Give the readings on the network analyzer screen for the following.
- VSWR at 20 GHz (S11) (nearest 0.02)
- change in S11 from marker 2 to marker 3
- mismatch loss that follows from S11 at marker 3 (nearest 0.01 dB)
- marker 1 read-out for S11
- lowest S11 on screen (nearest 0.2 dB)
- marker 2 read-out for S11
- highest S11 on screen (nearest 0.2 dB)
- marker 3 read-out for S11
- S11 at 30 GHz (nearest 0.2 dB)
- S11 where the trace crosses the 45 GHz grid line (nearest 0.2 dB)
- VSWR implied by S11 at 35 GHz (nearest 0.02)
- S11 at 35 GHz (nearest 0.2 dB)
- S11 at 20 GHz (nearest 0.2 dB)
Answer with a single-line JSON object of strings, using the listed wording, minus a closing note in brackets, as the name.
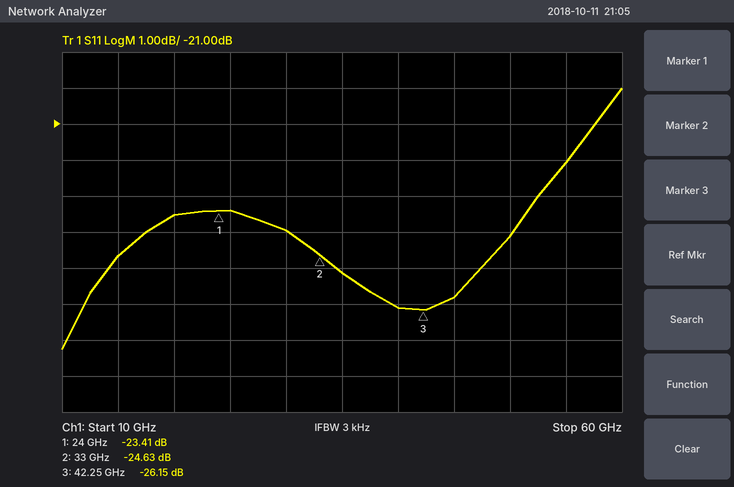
{"VSWR at 20 GHz (S11)": "1.14", "change in S11 from marker 2 to marker 3": "-1.52 dB", "mismatch loss that follows from S11 at marker 3": "0.01 dB", "marker 1 read-out for S11": "-23.41 dB", "lowest S11 on screen": "-27.2 dB", "marker 2 read-out for S11": "-24.63 dB", "highest S11 on screen": "-20.0 dB", "marker 3 read-out for S11": "-26.15 dB", "S11 at 30 GHz": "-24.0 dB", "S11 where the trace crosses the 45 GHz grid line": "-25.8 dB", "VSWR implied by S11 at 35 GHz": "1.12", "S11 at 35 GHz": "-25.2 dB", "S11 at 20 GHz": "-23.6 dB"}
